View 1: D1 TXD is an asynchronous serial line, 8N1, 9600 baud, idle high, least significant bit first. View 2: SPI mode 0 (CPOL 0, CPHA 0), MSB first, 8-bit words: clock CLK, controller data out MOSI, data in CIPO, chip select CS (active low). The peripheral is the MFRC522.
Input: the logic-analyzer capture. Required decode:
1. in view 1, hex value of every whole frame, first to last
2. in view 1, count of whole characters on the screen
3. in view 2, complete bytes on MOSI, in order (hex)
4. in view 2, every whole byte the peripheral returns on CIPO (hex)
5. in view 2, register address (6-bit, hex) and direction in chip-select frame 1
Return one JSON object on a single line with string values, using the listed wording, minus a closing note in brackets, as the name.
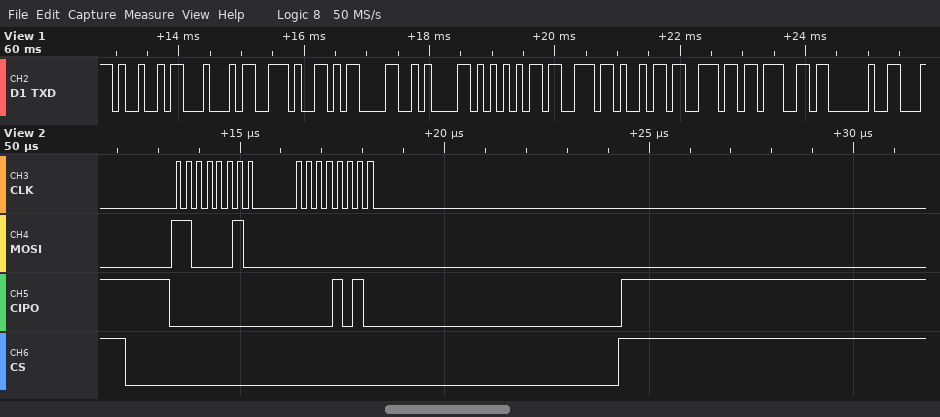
{"in view 1, hex value of every whole frame, first to last": "49 44 2E 0D 0A 55 73 69 6E 67 20", "in view 1, count of whole characters on the screen": "11", "in view 2, complete bytes on MOSI, in order": "C2 00", "in view 2, every whole byte the peripheral returns on CIPO": "00 0A", "in view 2, register address (6-bit, hex) and direction in chip-select frame 1": "0x21 read"}
